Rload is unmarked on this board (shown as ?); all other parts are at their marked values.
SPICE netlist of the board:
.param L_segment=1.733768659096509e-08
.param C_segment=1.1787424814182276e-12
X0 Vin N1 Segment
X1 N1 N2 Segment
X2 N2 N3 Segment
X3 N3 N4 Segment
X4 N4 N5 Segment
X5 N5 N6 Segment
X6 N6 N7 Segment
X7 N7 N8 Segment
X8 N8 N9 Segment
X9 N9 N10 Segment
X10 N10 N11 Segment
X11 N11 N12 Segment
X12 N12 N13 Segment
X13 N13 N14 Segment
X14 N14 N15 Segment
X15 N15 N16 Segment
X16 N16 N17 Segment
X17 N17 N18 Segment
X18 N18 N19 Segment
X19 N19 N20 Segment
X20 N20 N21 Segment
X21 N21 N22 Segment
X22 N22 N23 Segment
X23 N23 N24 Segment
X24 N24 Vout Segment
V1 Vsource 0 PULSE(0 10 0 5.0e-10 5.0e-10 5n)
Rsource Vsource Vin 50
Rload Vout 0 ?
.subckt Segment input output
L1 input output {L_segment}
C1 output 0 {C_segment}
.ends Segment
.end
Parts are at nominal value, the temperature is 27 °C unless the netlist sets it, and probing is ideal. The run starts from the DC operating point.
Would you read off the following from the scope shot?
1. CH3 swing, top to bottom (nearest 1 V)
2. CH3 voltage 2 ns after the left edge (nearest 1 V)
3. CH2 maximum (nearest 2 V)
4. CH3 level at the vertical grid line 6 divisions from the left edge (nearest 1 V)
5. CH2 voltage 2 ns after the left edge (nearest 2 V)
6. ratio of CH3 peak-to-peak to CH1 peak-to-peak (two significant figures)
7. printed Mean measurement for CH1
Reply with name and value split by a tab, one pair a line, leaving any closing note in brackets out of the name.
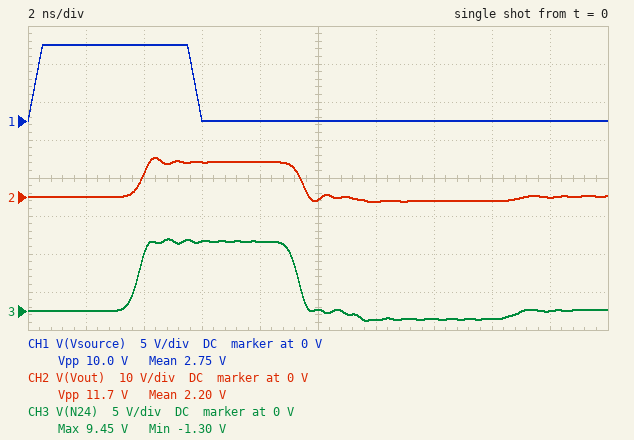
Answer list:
CH3 swing, top to bottom	11 V
CH3 voltage 2 ns after the left edge	0 V
CH2 maximum	10 V
CH3 level at the vertical grid line 6 divisions from the left edge	-1 V
CH2 voltage 2 ns after the left edge	0 V
ratio of CH3 peak-to-peak to CH1 peak-to-peak	1.1
printed Mean measurement for CH1	2.75 V
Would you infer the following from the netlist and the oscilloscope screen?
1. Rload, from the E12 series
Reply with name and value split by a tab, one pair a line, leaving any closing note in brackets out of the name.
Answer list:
Rload, from the E12 series	220 Ω
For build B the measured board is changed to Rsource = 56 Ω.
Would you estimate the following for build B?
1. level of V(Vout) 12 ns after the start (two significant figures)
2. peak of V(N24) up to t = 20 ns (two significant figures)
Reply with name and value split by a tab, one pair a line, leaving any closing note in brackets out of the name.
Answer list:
level of V(Vout) 12 ns after the start	-1.2 V
peak of V(N24) up to t = 20 ns	9.1 V
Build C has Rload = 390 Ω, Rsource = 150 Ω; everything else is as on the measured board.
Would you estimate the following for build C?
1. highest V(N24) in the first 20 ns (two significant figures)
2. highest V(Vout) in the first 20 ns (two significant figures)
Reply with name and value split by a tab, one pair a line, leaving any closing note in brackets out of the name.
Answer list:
highest V(N24) in the first 20 ns	7.0 V
highest V(Vout) in the first 20 ns	7.7 V
